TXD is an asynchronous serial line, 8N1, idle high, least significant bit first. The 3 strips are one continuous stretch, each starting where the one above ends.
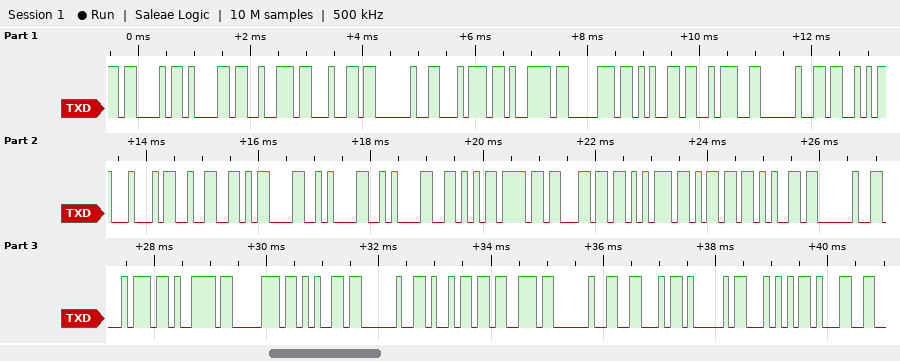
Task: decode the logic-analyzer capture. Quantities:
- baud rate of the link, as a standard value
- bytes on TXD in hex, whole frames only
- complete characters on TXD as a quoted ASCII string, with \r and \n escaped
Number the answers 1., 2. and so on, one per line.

1. 9600 baud
2. 43 61 72 64 20 74 79 70 65 3A 20 53 44 32 0D 0A 0A 56 6F 6C 75 6D 65 20 74 79 70 65 20 69 73 20 46 41 54 31
3. "Card type: SD2\r\n\nVolume type is FAT1"
